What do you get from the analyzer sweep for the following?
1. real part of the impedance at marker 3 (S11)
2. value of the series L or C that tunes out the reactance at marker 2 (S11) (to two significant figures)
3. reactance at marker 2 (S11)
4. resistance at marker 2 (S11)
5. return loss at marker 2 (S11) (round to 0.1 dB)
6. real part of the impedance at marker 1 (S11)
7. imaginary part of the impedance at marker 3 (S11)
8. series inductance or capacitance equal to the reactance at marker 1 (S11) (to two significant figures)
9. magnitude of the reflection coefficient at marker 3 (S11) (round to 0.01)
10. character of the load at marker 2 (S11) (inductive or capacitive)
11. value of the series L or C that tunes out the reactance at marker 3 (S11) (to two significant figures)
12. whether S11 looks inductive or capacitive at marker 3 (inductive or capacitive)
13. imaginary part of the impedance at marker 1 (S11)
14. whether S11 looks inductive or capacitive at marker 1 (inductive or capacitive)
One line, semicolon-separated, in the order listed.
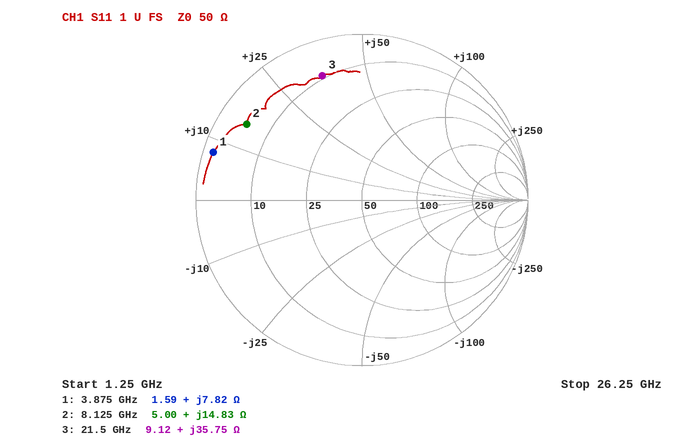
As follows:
9.12 Ω; 1.3 pF; +14.83 Ω; 5.00 Ω; 1.6 dB; 1.59 Ω; +35.75 Ω; 320 pH; 0.79; inductive; 210 fF; inductive; +7.82 Ω; inductive
